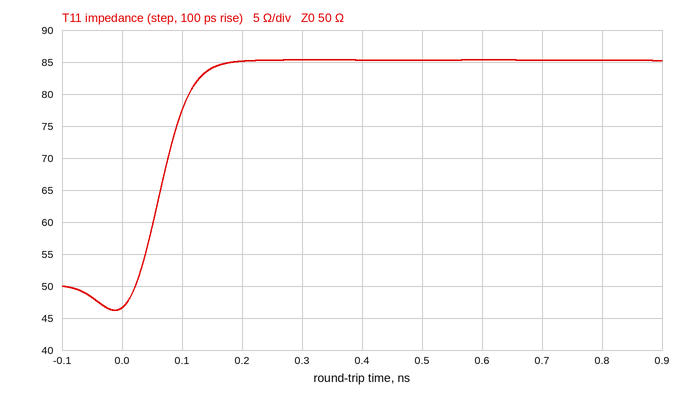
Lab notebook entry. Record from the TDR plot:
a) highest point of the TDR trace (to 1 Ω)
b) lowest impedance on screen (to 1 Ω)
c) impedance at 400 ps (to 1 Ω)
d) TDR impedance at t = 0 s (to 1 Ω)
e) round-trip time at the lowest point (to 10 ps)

85 Ω
46 Ω
85 Ω
47 Ω
-10 ps
